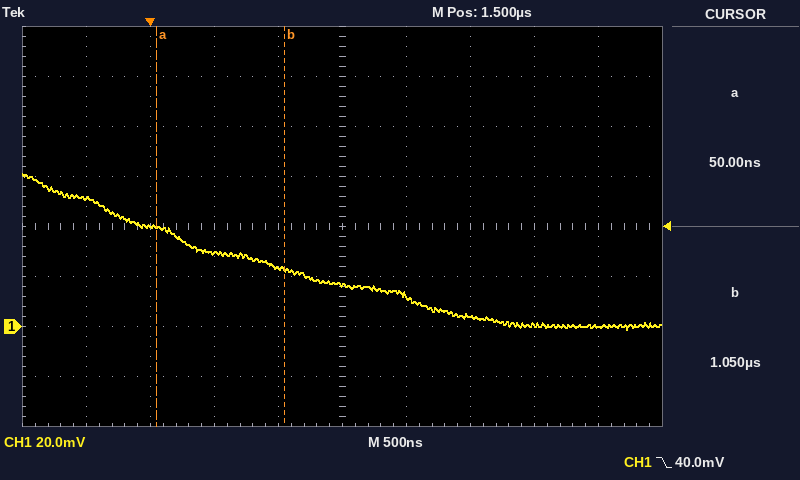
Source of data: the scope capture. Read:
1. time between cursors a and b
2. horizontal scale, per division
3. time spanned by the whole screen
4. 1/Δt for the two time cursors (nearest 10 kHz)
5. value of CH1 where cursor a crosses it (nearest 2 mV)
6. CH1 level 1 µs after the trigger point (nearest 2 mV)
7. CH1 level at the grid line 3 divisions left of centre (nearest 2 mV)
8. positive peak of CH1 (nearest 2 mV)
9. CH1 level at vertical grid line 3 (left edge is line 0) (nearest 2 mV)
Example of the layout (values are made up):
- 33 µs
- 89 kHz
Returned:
- 1.00 µs
- 500 ns
- 5 µs
- 1.00 MHz
- 40 mV
- 24 mV
- 40 mV
- 62 mV
- 30 mV
